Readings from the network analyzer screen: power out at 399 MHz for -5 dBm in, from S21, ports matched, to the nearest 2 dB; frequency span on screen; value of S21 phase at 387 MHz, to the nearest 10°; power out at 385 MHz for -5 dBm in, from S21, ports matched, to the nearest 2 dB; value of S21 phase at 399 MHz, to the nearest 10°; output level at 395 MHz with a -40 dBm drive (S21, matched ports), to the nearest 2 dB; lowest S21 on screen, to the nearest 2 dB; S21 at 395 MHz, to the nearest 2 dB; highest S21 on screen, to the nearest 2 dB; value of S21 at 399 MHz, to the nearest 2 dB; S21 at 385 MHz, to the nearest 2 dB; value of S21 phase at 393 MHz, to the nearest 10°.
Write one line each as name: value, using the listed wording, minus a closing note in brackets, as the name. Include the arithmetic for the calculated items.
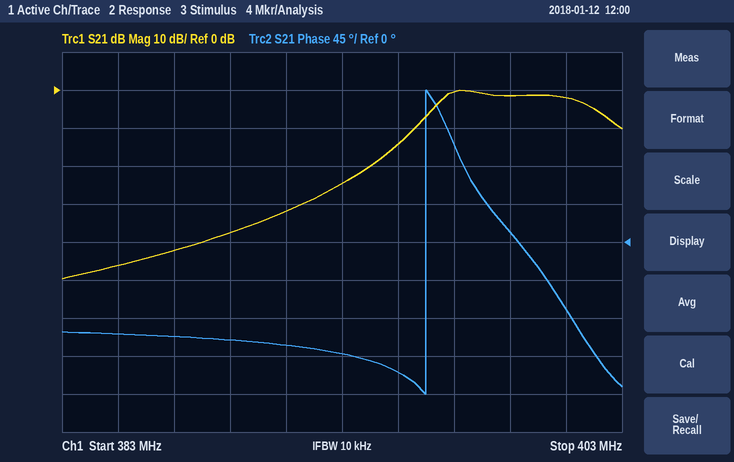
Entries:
power out at 399 MHz for -5 dBm in, from S21, ports matched, to the nearest 2 dB: -5 dBm + (-2 dB) = -6 dBm
frequency span on screen: 20 MHz
value of S21 phase at 387 MHz, to the nearest 10°: -110°
power out at 385 MHz for -5 dBm in, from S21, ports matched, to the nearest 2 dB: -5 dBm + (-46 dB) = -52 dBm
value of S21 phase at 399 MHz, to the nearest 10°: 10°
output level at 395 MHz with a -40 dBm drive (S21, matched ports), to the nearest 2 dB: -40 dBm + (-14 dB) = -54 dBm
lowest S21 on screen, to the nearest 2 dB: -50 dB
S21 at 395 MHz, to the nearest 2 dB: -14 dB
highest S21 on screen, to the nearest 2 dB: 0 dB
value of S21 at 399 MHz, to the nearest 2 dB: -2 dB
S21 at 385 MHz, to the nearest 2 dB: -46 dB
value of S21 phase at 393 MHz, to the nearest 10°: -130°
